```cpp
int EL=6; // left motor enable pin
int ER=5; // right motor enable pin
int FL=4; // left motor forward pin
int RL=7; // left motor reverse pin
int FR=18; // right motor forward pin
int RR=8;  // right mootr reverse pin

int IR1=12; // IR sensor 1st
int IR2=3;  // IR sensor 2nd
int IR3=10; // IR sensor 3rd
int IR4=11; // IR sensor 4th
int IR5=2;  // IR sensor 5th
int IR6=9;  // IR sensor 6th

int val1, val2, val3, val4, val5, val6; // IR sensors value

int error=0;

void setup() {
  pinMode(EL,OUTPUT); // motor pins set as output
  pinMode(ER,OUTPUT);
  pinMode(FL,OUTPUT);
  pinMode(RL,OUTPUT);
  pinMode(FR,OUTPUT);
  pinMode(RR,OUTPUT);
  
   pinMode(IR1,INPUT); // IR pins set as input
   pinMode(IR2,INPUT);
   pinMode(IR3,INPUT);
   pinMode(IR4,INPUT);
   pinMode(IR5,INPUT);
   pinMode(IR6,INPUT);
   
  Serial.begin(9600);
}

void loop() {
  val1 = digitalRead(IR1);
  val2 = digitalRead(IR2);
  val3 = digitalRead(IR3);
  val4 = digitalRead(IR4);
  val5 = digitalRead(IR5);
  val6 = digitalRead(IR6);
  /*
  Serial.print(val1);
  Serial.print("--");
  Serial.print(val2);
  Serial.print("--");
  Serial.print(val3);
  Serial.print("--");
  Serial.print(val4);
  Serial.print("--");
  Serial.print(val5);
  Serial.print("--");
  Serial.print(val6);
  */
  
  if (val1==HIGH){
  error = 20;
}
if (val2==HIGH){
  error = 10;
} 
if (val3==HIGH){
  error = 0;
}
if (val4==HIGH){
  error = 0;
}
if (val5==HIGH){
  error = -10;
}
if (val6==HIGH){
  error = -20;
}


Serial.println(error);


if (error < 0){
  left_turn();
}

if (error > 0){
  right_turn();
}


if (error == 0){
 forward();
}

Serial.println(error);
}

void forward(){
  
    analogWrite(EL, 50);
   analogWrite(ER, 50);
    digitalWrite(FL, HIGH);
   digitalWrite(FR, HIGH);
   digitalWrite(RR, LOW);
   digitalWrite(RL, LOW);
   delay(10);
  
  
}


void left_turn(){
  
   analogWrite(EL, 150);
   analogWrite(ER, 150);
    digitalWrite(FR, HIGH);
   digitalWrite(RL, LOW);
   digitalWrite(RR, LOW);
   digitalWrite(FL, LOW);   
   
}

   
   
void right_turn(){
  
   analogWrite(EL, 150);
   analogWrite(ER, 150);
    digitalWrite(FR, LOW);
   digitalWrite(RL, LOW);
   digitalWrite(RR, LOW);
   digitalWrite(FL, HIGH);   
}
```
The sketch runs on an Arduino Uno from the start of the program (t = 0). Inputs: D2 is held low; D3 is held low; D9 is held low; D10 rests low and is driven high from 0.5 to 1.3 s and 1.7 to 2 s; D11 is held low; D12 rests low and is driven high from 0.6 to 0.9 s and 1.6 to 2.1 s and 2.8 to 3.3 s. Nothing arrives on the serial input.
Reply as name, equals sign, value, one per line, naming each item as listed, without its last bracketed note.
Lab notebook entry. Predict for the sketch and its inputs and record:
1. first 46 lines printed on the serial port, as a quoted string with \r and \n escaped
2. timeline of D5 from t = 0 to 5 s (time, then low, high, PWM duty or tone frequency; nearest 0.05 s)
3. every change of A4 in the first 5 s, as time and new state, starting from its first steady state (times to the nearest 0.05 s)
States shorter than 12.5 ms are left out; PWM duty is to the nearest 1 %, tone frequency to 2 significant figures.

first 46 lines printed on the serial port, as a quoted string with \r and \n escaped = "0\r\n0\r\n0\r\n0\r\n0\r\n0\r\n0\r\n0\r\n0\r\n0\r\n0\r\n0\r\n0\r\n0\r\n0\r\n0\r\n0\r\n0\r\n0\r\n0\r\n0\r\n0\r\n0\r\n0\r\n0\r\n0\r\n0\r\n0\r\n0\r\n0\r\n0\r\n0\r\n0\r\n0\r\n0\r\n0\r\n0\r\n0\r\n0\r\n0\r\n0\r\n0\r\n0\r\n0\r\n0\r\n0\r\n"
timeline of D5 from t = 0 to 5 s = 0 s PWM 20 %; 1.6 s PWM 59 %; 1.7 s PWM 20 %; 2 s PWM 59 %
every change of A4 in the first 5 s, as time and new state, starting from its first steady state = 0 s high; 1.6 s low; 1.7 s high; 2 s low
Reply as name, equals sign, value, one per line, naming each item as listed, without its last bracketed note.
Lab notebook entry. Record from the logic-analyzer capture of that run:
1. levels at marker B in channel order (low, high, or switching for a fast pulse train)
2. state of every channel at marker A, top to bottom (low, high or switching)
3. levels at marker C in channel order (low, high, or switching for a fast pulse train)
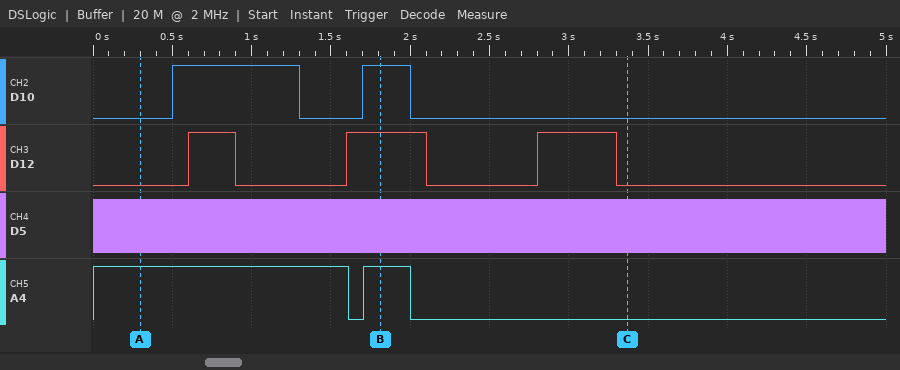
levels at marker B in channel order = D10 high, D12 high, D5 switching, A4 high
state of every channel at marker A, top to bottom = D10 low, D12 low, D5 switching, A4 high
levels at marker C in channel order = D10 low, D12 low, D5 switching, A4 low
